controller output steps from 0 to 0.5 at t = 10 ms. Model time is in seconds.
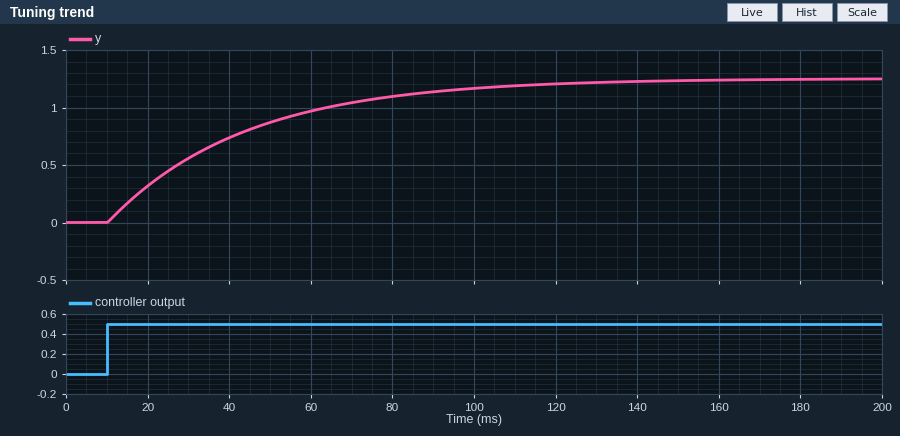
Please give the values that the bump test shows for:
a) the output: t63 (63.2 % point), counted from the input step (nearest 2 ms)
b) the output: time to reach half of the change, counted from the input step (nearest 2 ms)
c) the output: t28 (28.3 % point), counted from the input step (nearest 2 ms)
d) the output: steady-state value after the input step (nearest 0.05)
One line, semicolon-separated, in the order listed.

34 ms; 24 ms; 12 ms; 1.25
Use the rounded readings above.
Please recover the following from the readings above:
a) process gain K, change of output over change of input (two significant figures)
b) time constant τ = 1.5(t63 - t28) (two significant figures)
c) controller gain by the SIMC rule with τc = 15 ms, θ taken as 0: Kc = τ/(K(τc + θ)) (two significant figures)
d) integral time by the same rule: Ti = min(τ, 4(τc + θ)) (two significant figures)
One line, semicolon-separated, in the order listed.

2.5; 33 ms; 0.88; 33 ms
